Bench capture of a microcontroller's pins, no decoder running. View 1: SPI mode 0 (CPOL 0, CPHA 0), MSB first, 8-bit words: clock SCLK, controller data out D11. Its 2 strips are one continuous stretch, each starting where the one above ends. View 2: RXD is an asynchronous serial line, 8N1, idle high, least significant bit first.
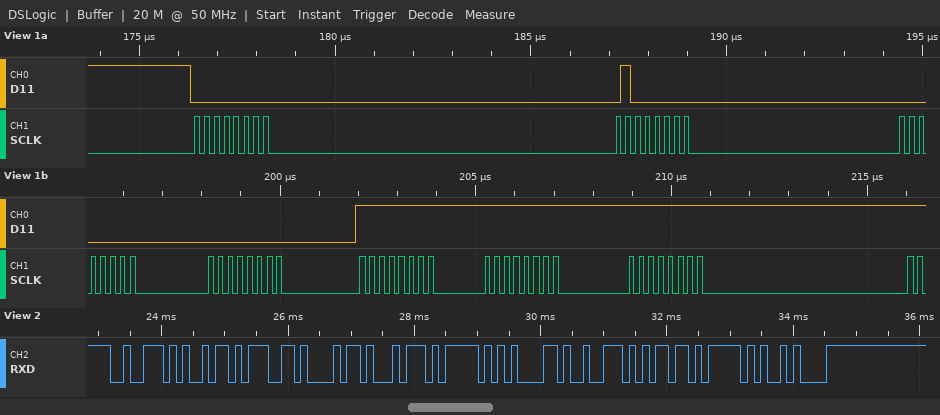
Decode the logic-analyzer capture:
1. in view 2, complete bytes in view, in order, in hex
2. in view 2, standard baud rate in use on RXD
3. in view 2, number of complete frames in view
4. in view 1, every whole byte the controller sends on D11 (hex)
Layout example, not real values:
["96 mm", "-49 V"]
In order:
["72 69 67 68 74 5F 61 72 6D 5F 0A", "9600 baud", "11", "0x00 0x40 0x00 0x00 0xFF 0xFF 0xFF"]
